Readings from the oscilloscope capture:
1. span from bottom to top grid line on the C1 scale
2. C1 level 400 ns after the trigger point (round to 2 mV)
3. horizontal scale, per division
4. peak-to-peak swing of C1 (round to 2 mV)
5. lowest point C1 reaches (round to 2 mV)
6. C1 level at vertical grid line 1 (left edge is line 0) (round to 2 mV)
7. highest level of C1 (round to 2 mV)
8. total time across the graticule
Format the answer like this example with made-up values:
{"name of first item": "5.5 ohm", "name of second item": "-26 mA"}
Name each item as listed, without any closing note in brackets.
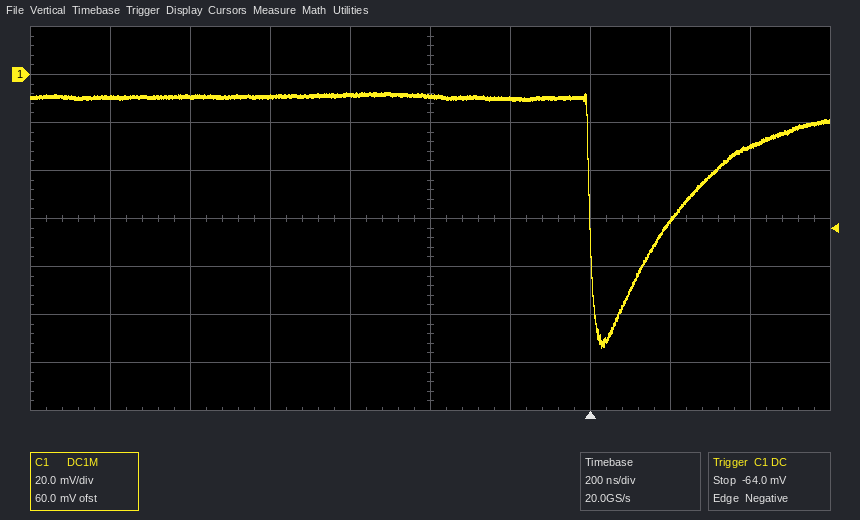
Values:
{"span from bottom to top grid line on the C1 scale": "160 mV", "C1 level 400 ns after the trigger point": "-30 mV", "horizontal scale, per division": "200 ns", "peak-to-peak swing of C1": "106 mV", "lowest point C1 reaches": "-114 mV", "C1 level at vertical grid line 1 (left edge is line 0)": "-10 mV", "highest level of C1": "-8 mV", "total time across the graticule": "2 µs"}
